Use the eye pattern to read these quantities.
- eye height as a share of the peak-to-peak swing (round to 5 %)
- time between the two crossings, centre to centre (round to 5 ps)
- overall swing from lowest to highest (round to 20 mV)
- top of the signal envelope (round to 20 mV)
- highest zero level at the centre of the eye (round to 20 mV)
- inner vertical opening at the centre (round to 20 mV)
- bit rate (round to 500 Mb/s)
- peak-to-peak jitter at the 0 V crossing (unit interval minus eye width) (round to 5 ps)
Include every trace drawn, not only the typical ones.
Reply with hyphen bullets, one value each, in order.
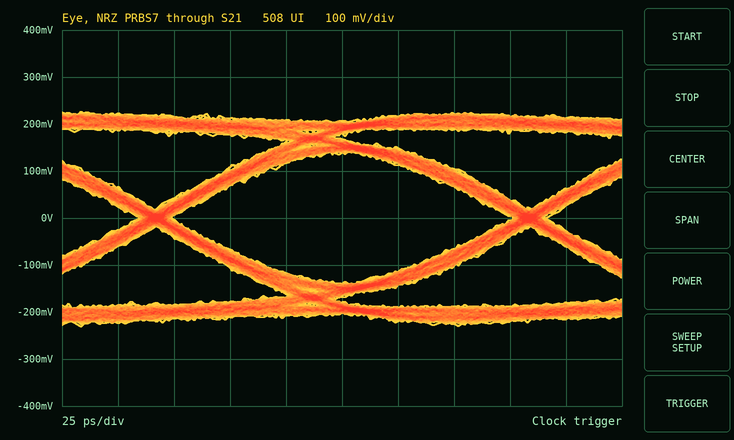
- 60 %
- 165 ps
- 460 mV
- 220 mV
- -140 mV
- 280 mV
- 6.0 Gb/s
- 15 ps
